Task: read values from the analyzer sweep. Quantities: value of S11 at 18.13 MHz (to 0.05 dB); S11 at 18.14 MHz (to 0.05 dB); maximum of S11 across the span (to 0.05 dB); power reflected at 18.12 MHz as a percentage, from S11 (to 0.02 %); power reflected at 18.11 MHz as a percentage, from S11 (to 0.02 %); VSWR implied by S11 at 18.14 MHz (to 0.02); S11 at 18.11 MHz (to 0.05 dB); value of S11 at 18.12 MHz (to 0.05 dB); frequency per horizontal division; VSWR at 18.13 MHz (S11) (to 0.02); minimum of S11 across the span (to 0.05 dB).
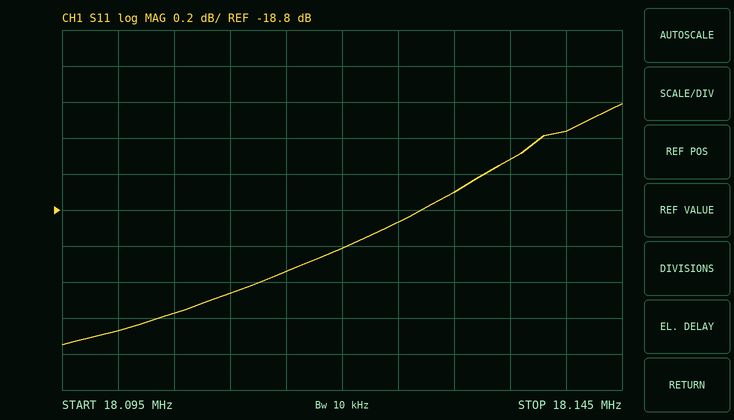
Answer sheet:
-18.70 dB
-18.35 dB
-18.20 dB
1.26 %
1.18 %
1.28
-19.25 dB
-19.00 dB
5 kHz
1.26
-19.55 dB
